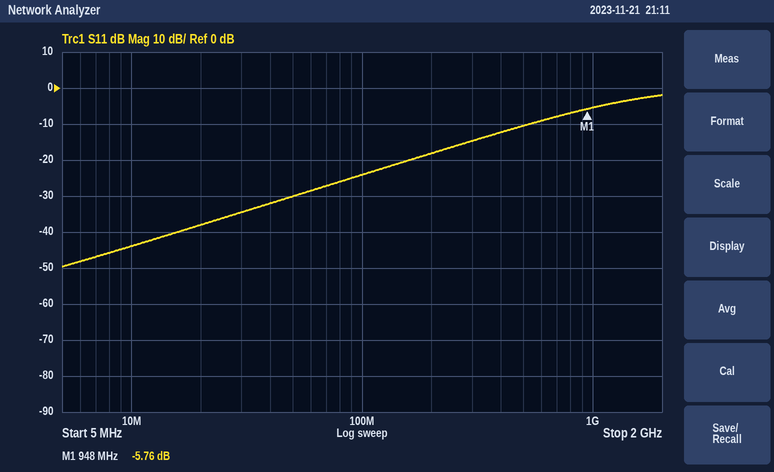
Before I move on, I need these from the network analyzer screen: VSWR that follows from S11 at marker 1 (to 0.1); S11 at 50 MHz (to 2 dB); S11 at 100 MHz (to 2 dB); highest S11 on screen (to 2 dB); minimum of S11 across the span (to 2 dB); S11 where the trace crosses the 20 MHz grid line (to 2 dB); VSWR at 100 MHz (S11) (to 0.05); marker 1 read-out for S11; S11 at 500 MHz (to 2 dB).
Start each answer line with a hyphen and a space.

- 3.1
- -30 dB
- -24 dB
- -2 dB
- -50 dB
- -38 dB
- 1.15
- -5.76 dB
- -10 dB
